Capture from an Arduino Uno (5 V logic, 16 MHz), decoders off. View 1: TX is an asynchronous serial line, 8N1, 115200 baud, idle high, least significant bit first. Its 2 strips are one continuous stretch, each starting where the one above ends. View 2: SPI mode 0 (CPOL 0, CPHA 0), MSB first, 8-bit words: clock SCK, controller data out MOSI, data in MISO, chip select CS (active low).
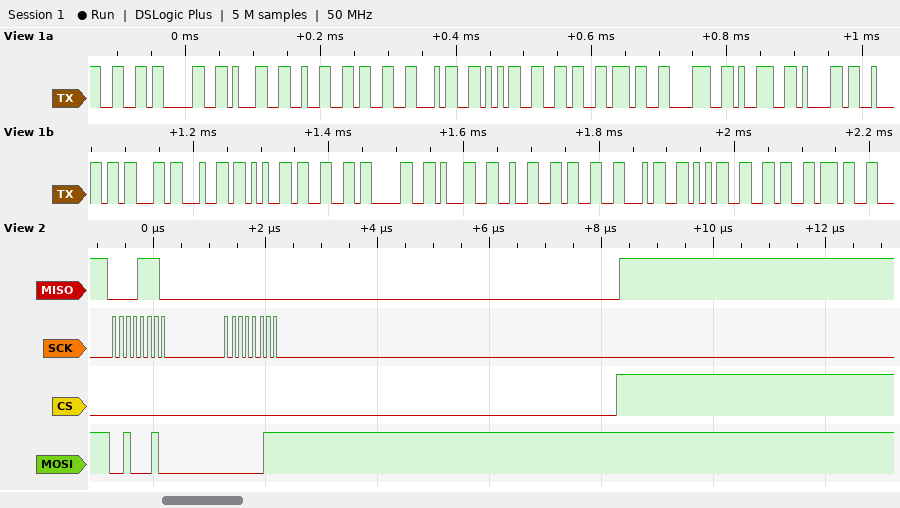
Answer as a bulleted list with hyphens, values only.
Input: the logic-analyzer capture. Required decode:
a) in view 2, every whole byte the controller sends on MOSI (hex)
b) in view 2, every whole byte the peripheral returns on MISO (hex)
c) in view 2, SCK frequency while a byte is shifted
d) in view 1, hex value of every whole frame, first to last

- 22 03
- 0E 00
- 8 MHz
- 0x66 0x30 0x31 0x32 0x33 0x34 0x35 0x36 0x37 0x38 0x39 0x61 0x62 0x63 0x64 0x65 0x66 0x30 0x31 0x32 0x33 0x34 0x35 0x36 0x37
